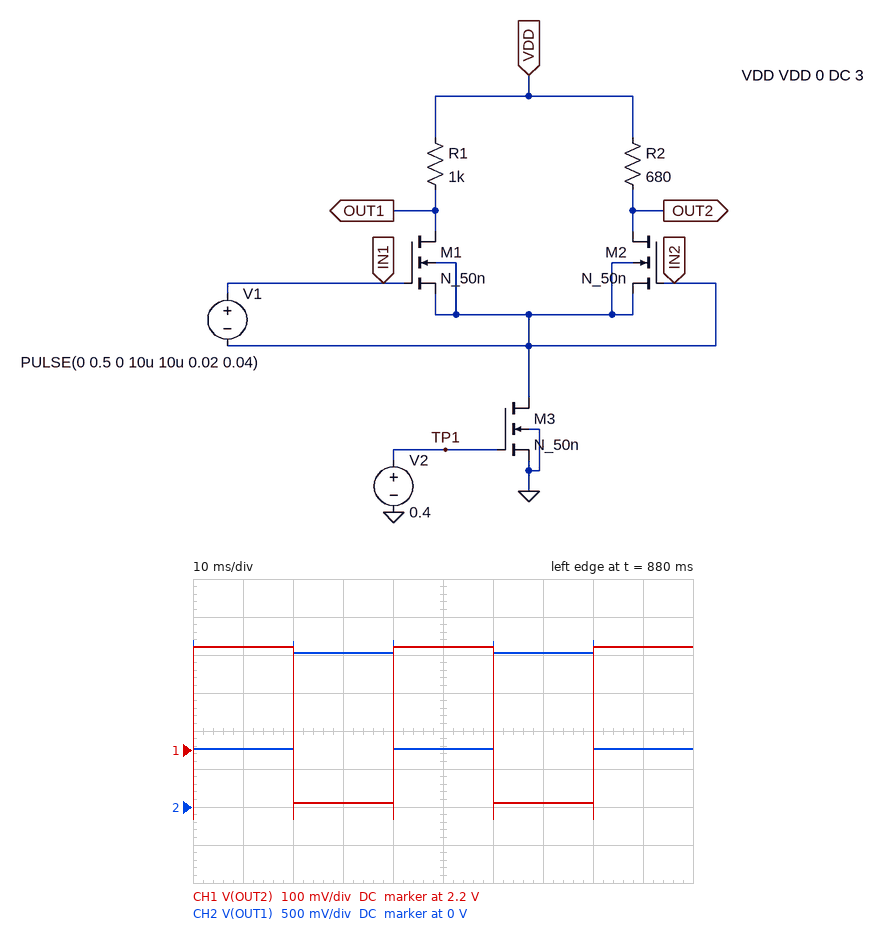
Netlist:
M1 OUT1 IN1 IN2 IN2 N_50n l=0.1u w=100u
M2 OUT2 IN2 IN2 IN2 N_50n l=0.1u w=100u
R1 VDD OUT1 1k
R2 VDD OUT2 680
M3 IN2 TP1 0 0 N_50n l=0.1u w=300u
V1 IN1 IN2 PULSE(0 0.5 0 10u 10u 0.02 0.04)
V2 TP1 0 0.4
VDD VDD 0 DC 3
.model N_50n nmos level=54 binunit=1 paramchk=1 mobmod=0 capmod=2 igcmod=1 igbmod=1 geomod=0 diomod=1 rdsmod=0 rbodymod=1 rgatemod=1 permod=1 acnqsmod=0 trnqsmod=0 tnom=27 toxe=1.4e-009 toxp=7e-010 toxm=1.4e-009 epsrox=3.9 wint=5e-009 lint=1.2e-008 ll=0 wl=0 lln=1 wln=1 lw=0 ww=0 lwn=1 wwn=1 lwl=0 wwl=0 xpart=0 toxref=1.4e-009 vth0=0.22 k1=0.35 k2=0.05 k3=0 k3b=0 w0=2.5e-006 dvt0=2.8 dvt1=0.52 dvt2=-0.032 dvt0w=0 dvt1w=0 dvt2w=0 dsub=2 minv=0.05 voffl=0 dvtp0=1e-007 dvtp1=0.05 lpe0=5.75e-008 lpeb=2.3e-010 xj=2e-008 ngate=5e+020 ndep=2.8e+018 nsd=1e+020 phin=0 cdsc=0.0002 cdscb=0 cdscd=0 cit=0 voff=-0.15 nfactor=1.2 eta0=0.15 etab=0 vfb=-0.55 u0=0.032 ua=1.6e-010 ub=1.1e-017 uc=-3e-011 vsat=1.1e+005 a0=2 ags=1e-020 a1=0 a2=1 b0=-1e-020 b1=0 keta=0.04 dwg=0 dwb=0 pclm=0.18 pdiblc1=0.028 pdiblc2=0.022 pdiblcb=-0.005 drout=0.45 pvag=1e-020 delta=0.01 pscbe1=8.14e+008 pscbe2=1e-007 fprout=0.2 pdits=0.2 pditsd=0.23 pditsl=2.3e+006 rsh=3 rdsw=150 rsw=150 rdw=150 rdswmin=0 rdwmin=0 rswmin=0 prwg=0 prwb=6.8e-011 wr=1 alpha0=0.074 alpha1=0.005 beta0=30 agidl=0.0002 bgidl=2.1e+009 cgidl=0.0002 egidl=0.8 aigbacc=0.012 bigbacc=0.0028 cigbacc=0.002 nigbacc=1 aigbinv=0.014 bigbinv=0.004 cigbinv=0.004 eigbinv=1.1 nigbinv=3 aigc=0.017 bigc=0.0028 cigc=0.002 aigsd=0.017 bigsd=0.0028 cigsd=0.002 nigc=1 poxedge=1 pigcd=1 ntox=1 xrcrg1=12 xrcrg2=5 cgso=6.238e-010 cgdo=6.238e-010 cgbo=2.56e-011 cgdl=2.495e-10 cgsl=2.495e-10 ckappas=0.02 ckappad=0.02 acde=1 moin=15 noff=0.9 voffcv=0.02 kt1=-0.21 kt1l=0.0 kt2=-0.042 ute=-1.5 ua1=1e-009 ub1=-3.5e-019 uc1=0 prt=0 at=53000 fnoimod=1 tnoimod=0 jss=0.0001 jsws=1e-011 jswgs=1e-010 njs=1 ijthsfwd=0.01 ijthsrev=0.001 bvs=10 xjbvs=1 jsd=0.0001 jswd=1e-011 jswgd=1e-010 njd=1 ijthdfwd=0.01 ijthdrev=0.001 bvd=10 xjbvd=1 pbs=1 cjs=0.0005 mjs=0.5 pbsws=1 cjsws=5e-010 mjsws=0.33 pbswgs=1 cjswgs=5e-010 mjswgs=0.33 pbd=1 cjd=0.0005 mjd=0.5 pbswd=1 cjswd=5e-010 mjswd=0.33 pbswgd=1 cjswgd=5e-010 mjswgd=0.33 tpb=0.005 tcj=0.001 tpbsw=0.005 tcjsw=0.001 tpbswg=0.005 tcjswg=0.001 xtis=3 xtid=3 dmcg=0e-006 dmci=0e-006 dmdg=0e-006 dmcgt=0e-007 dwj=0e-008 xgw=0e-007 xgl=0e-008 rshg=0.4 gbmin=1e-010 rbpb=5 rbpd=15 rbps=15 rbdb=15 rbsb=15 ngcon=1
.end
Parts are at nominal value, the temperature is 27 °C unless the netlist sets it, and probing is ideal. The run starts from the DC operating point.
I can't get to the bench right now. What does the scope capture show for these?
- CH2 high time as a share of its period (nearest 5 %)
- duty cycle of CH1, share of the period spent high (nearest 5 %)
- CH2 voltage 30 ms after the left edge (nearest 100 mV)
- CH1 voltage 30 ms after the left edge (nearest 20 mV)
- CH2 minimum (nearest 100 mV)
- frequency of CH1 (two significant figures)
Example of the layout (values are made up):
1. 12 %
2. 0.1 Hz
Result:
1. 50 %
2. 50 %
3. 2.0 V
4. 2.06 V
5. 800 mV
6. 25 Hz
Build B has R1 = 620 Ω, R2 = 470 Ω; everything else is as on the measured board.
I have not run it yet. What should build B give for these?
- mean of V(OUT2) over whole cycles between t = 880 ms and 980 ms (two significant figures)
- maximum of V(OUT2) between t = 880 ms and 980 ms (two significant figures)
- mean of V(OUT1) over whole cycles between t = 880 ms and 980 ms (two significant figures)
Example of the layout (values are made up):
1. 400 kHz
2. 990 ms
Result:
1. 2.5 V
2. 2.7 V
3. 1.8 V
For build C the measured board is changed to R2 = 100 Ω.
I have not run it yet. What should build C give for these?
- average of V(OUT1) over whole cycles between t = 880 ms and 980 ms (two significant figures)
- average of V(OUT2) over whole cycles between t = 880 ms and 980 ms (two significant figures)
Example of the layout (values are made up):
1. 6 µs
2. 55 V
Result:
1. 1.8 V
2. 2.8 V
